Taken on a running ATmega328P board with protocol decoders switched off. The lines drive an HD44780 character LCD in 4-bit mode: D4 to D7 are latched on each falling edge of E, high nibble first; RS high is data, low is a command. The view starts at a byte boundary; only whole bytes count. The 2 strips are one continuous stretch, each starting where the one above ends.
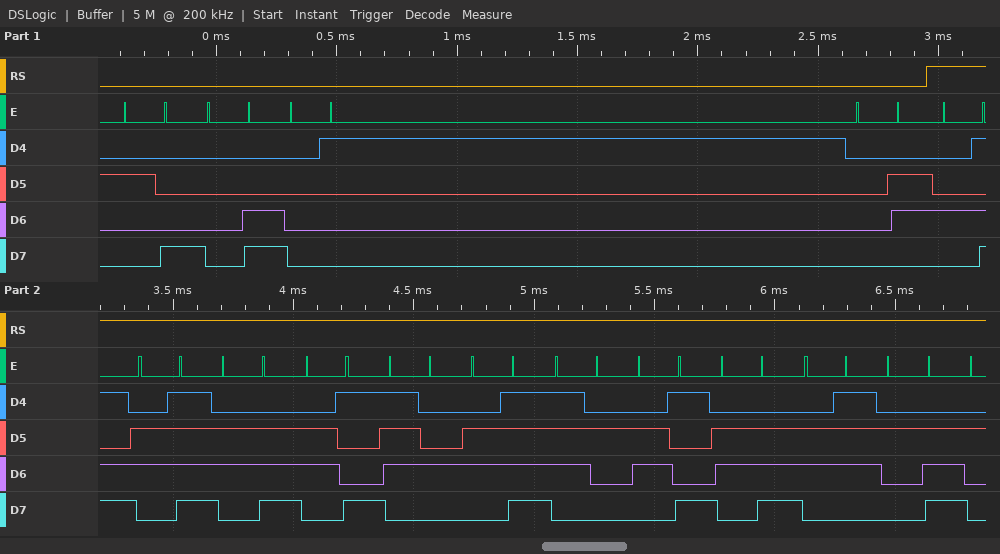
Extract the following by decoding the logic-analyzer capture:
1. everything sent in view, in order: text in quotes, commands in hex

0x28 0x0C 0x01 0x06 "Monitoring."
